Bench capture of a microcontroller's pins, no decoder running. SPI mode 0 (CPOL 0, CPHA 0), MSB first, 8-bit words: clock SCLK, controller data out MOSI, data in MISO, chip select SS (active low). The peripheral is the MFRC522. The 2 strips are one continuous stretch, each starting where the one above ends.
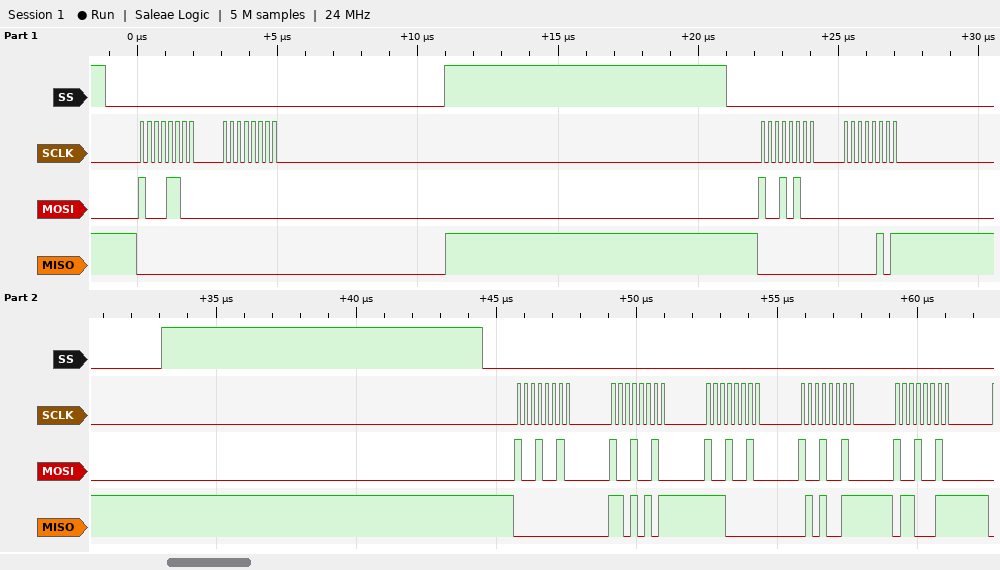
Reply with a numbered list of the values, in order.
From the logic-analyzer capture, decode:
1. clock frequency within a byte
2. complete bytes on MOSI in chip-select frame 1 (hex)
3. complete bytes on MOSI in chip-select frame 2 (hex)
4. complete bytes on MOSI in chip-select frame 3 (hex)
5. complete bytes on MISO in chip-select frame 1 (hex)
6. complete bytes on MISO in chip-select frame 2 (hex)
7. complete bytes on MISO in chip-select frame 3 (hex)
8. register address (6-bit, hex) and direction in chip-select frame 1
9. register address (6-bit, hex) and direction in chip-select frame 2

1. 4 MHz
2. 8C 00
3. 94 00
4. 92 92 92 92 92
5. 00 00
6. 00 05
7. 00 D5 E0 53 63
8. 0x06 read
9. 0x0A read
